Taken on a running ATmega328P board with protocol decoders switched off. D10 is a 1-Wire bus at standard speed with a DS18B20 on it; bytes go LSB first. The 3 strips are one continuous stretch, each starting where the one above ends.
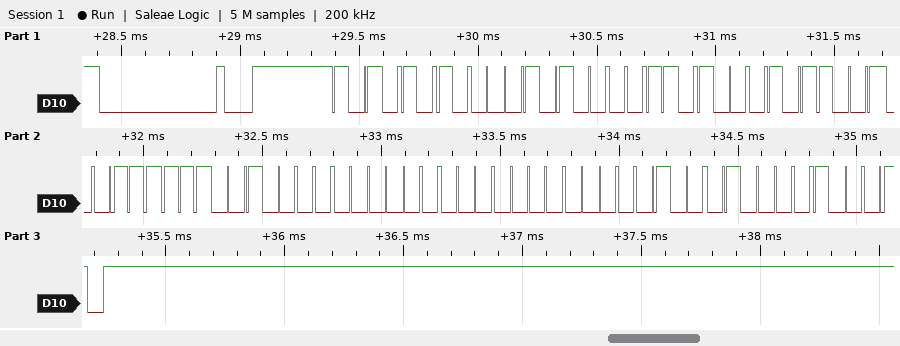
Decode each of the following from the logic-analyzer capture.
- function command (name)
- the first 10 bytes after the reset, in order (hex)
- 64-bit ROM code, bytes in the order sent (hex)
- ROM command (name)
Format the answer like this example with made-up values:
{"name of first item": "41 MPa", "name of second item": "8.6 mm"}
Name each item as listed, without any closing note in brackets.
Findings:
{"function command": "Convert T", "the first 10 bytes after the reset, in order": "55 28 2C 9A FC 04 00 00 22 44", "64-bit ROM code, bytes in the order sent": "28 2C 9A FC 04 00 00 22", "ROM command": "Match ROM"}
